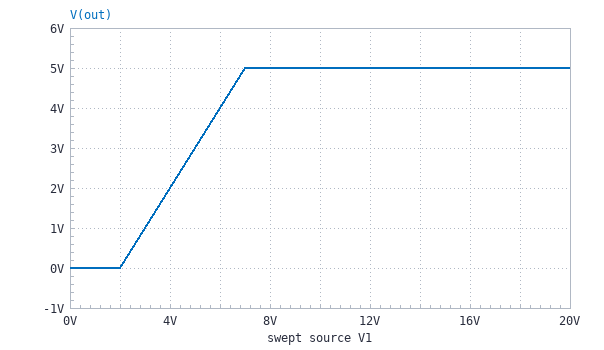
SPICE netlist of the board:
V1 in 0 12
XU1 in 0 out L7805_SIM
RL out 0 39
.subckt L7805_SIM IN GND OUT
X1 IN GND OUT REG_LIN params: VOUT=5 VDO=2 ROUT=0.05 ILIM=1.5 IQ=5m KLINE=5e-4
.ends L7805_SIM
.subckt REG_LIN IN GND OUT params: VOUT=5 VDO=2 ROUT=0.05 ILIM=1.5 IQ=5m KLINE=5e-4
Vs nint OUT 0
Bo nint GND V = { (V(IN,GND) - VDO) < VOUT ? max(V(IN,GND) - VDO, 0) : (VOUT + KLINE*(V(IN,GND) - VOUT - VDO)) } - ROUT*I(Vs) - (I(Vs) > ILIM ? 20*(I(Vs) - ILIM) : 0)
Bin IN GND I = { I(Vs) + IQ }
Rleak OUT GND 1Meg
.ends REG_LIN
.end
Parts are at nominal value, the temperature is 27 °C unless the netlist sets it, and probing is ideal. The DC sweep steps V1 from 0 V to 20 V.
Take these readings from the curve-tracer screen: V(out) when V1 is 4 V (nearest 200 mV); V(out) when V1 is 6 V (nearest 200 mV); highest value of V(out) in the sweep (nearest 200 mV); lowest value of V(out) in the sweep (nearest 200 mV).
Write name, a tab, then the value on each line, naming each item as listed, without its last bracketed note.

V(out) when V1 is 4 V	2.0 V
V(out) when V1 is 6 V	4.0 V
highest value of V(out) in the sweep	5.0 V
lowest value of V(out) in the sweep	0 V
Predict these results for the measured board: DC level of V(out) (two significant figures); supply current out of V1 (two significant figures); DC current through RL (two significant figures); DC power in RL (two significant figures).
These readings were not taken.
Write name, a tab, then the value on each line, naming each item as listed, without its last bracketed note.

DC level of V(out)	5.0 V
supply current out of V1	130 mA
DC current through RL	130 mA
DC power in RL	640 mW
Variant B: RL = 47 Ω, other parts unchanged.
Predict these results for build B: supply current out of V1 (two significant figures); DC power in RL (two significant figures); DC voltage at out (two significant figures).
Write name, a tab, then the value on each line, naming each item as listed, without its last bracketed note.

supply current out of V1	110 mA
DC power in RL	530 mW
DC voltage at out	5.0 V
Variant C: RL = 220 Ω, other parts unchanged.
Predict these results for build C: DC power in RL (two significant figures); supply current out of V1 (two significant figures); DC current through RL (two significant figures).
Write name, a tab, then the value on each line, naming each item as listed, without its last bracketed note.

DC power in RL	110 mW
supply current out of V1	28 mA
DC current through RL	23 mA
